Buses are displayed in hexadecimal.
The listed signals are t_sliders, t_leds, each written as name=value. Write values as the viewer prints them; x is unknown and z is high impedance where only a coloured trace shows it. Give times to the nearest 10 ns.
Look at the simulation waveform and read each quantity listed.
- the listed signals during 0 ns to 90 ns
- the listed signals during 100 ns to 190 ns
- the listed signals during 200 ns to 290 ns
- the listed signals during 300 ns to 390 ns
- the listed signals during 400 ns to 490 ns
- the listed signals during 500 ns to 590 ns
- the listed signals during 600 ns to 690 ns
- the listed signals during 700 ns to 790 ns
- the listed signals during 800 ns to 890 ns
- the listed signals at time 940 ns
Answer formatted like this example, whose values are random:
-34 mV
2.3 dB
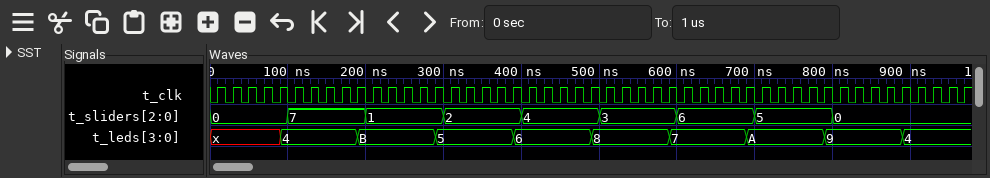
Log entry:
t_sliders=0, t_leds=x
t_sliders=7, t_leds=4
t_sliders=1, t_leds=B
t_sliders=2, t_leds=5
t_sliders=4, t_leds=6
t_sliders=3, t_leds=8
t_sliders=6, t_leds=7
t_sliders=5, t_leds=A
t_sliders=0, t_leds=9
t_sliders=0, t_leds=4
